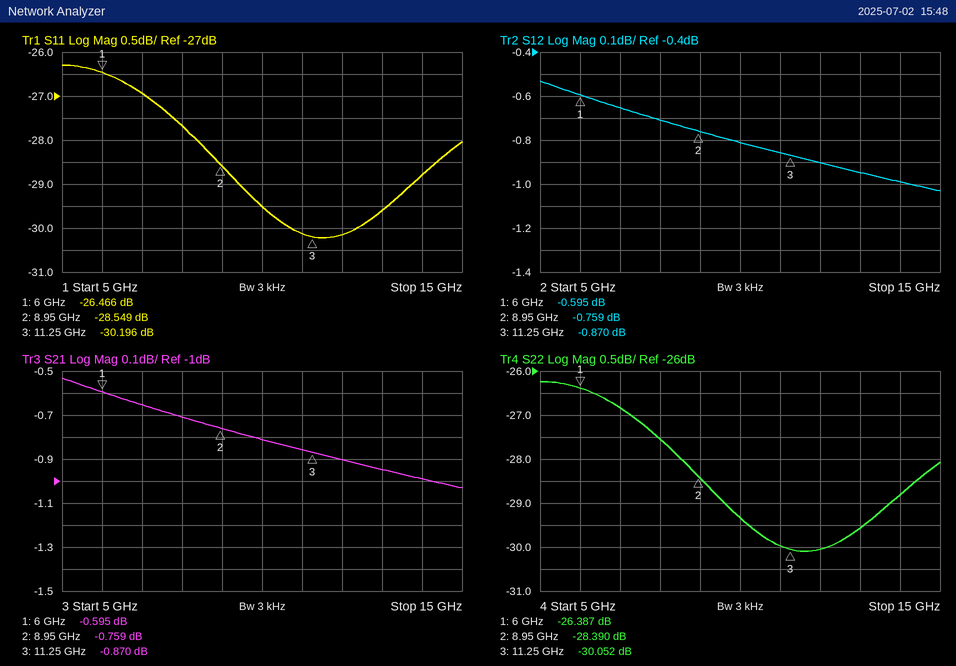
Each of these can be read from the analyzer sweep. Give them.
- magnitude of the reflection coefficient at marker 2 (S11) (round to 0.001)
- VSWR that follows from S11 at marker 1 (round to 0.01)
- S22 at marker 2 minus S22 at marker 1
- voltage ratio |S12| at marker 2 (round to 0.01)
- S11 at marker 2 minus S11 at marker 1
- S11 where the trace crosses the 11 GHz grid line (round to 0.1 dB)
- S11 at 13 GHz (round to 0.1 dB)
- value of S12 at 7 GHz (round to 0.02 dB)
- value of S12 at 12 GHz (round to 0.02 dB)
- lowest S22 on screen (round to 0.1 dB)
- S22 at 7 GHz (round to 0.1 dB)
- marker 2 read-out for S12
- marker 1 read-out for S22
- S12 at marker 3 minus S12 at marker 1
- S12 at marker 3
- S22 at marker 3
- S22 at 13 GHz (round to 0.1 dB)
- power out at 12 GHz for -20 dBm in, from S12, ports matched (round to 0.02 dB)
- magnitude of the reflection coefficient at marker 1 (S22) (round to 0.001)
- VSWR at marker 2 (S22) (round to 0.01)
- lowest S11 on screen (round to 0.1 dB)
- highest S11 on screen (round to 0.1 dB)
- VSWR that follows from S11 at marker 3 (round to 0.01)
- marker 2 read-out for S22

0.037
1.10
-2.003 dB
0.92
-2.083 dB
-30.1 dB
-29.6 dB
-0.66 dB
-0.90 dB
-30.1 dB
-26.8 dB
-0.759 dB
-26.387 dB
-0.275 dB
-0.870 dB
-30.052 dB
-29.6 dB
-20.90 dBm
0.048
1.08
-30.2 dB
-26.3 dB
1.06
-28.390 dB
